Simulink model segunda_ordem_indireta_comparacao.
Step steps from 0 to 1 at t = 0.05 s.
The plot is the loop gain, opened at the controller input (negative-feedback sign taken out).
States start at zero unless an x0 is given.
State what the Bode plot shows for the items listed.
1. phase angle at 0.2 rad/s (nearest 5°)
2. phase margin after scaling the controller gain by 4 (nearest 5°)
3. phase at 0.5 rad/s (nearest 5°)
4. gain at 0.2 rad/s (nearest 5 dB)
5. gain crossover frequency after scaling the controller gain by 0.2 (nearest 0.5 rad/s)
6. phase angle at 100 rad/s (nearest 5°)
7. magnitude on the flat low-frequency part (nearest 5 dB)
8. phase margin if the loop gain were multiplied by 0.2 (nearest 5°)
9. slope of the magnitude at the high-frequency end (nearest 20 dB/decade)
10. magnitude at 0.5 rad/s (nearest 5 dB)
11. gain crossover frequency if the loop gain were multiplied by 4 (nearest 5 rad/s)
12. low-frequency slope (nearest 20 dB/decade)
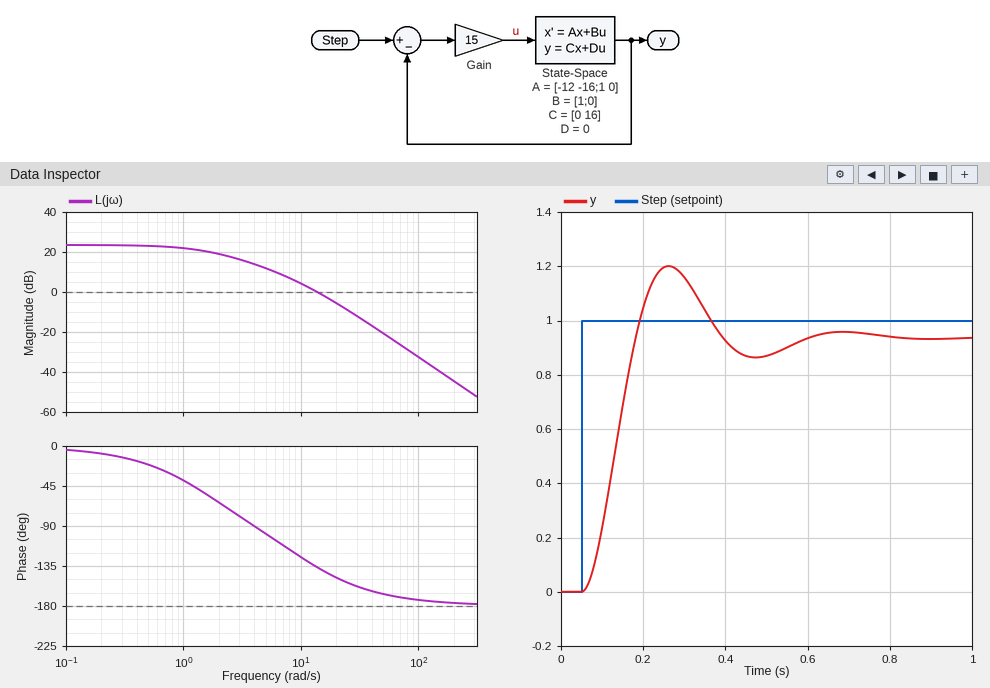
-10°
20°
-20°
25 dB
4.0 rad/s
-175°
25 dB
90°
-40 dB/decade
25 dB
30 rad/s
0 dB/decade
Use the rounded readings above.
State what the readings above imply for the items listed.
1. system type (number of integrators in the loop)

0
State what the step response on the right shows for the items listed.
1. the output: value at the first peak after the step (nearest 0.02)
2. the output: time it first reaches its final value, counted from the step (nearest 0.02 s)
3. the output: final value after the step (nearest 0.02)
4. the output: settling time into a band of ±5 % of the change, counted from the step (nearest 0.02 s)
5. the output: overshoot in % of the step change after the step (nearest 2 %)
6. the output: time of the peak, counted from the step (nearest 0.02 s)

1.20
0.14 s
0.94
0.48 s
28 %
0.22 s
